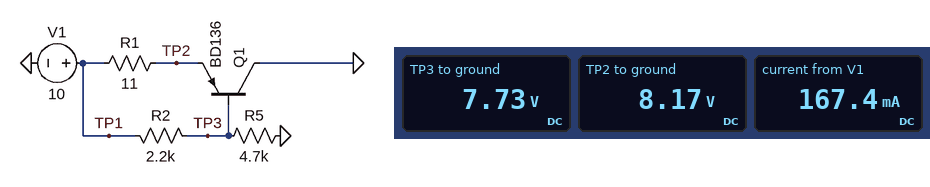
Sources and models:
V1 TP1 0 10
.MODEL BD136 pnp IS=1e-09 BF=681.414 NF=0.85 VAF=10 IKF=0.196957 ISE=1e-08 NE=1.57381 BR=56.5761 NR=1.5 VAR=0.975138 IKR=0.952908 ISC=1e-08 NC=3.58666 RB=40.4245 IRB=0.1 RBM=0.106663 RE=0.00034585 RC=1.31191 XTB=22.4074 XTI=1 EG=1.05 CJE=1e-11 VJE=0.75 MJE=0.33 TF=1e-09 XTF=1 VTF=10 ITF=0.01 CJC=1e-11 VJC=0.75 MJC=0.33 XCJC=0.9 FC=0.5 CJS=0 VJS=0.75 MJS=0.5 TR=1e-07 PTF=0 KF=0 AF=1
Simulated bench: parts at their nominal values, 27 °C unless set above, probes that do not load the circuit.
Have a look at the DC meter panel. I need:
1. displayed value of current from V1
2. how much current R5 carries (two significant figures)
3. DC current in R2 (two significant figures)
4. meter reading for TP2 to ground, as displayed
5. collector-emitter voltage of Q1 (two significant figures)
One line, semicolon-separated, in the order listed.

167.4 mA; 1.6 mA; 1.0 mA; 8.17 V; -8.2 V
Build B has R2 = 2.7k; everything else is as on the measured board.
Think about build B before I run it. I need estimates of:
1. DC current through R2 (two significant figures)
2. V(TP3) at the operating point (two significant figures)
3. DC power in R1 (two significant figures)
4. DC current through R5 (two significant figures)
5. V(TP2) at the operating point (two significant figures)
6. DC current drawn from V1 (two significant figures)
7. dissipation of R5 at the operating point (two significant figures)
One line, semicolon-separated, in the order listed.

910 µA; 7.5 V; 370 mW; 1.6 mA; 8.0 V; 180 mA; 12 mW
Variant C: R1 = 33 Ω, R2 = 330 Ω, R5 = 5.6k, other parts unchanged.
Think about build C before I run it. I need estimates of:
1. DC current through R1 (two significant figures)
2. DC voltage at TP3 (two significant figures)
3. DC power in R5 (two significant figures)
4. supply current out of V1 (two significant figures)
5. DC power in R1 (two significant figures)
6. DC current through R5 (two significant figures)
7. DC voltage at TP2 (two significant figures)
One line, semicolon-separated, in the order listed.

6.3 mA; 9.5 V; 16 mW; 7.9 mA; 1.3 mW; 1.7 mA; 9.8 V
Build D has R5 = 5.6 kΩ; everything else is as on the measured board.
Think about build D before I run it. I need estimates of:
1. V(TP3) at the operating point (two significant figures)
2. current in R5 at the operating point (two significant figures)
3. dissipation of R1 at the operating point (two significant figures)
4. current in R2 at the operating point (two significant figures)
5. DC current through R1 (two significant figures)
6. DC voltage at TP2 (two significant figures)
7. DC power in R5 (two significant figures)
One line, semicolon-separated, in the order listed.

8.0 V; 1.4 mA; 230 mW; 920 µA; 140 mA; 8.4 V; 11 mW
